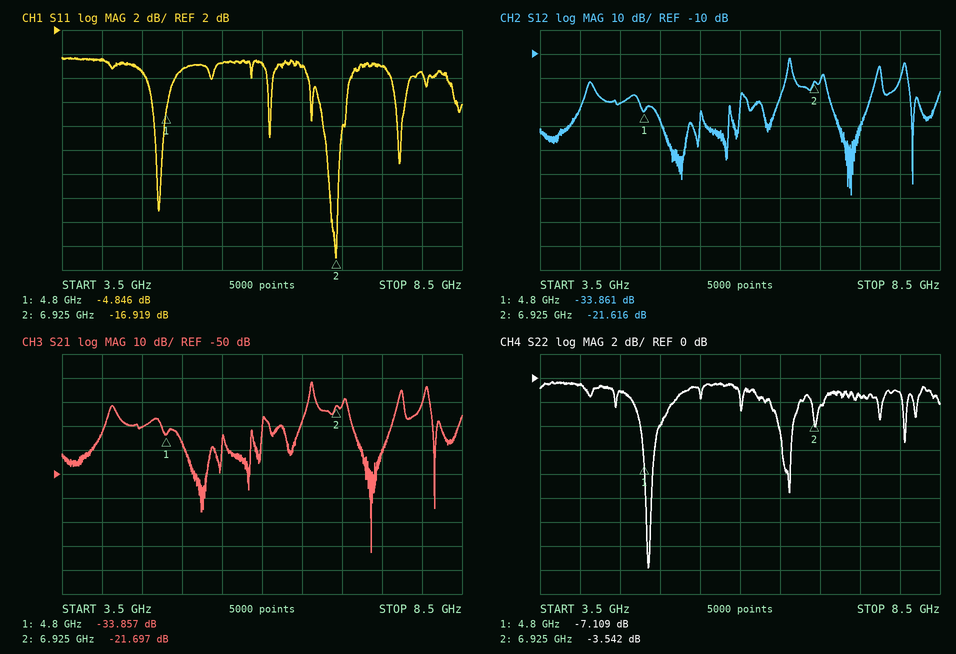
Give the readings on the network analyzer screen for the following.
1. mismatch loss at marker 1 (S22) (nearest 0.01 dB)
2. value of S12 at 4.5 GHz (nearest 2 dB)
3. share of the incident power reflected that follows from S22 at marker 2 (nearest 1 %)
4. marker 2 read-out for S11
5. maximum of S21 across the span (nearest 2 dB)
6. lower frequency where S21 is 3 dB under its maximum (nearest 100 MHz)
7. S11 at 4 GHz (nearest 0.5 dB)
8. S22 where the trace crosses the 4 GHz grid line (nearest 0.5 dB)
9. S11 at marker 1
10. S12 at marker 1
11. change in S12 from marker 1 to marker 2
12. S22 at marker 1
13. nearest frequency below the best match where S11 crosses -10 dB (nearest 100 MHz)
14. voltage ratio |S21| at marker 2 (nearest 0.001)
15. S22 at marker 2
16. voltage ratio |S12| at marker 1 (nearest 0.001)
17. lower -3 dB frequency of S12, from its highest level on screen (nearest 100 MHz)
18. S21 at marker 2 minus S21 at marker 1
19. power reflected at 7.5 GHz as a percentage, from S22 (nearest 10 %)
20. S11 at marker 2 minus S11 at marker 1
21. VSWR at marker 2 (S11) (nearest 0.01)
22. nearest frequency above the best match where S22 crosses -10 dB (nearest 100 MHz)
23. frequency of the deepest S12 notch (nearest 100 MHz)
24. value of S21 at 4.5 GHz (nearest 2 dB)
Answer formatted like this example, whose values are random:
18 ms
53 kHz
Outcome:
0.94 dB
-30 dB
44 %
-16.919 dB
-12 dB
6.6 GHz
-0.5 dB
-0.5 dB
-4.846 dB
-33.861 dB
12.245 dB
-7.109 dB
6.8 GHz
0.082
-3.542 dB
0.020
6.6 GHz
12.160 dB
70 %
-12.073 dB
1.33
4.9 GHz
7.4 GHz
-30 dB
